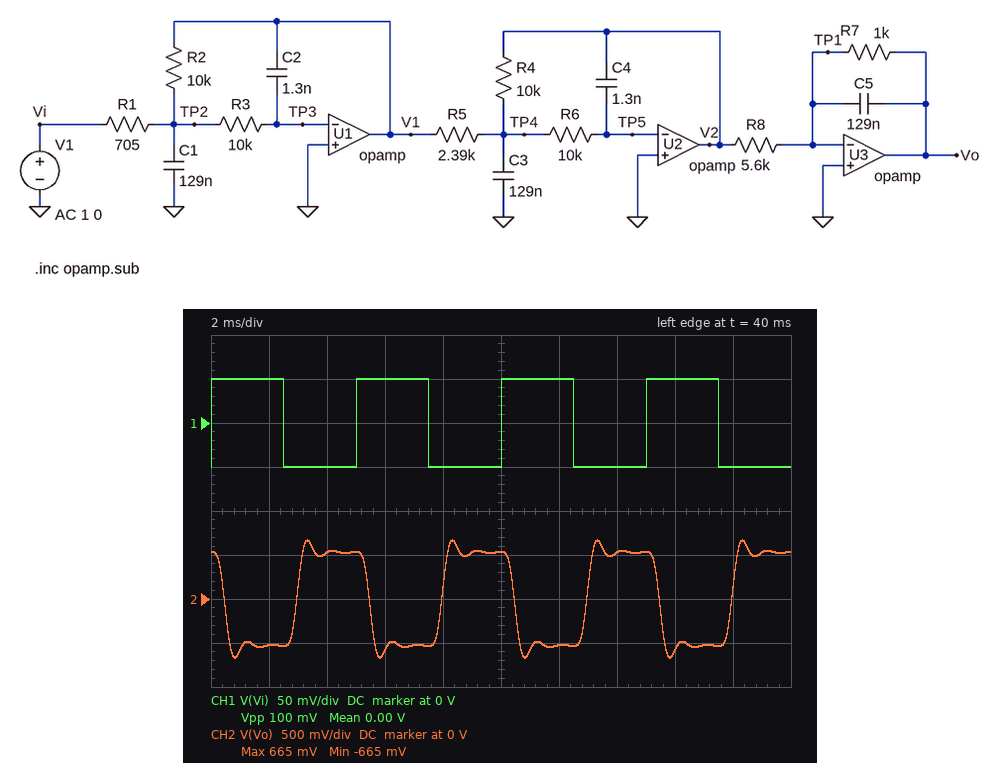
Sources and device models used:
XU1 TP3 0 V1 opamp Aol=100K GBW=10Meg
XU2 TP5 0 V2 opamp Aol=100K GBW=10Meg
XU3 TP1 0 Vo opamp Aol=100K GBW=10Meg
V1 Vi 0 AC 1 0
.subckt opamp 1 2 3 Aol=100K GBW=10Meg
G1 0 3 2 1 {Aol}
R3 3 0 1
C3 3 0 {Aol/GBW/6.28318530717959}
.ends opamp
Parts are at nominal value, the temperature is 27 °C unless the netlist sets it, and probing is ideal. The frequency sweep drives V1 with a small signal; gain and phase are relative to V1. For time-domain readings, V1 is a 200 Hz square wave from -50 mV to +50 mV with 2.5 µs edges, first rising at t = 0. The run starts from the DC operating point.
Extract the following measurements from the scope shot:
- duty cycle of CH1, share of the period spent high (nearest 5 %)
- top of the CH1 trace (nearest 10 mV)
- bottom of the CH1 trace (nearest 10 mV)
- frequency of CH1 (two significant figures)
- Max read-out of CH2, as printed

50 %
50 mV
-50 mV
200 Hz
665 mV
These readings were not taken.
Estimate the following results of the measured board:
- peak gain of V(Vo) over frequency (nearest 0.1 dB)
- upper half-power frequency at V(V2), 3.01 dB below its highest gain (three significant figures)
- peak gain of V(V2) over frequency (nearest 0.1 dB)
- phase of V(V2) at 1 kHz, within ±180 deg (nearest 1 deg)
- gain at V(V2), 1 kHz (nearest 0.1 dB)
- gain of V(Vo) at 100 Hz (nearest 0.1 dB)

20.5 dB
1.31 kHz
37.1 dB
-132 deg
37.1 dB
20.5 dB
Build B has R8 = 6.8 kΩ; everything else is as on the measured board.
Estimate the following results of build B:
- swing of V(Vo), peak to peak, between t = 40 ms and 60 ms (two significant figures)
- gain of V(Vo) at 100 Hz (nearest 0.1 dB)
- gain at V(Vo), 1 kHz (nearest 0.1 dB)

1.1 V
18.8 dB
18.2 dB
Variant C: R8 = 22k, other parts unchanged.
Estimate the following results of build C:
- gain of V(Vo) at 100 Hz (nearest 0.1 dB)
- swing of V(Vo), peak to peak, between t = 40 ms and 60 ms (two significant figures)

8.6 dB
340 mV
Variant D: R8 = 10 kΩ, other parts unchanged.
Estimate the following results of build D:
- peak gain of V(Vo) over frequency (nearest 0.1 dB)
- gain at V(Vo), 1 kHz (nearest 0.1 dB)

15.5 dB
14.9 dB
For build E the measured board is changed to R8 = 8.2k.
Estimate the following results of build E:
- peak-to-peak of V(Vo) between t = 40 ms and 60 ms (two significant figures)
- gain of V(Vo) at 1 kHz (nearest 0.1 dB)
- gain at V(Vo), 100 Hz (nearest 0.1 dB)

910 mV
16.6 dB
17.2 dB
